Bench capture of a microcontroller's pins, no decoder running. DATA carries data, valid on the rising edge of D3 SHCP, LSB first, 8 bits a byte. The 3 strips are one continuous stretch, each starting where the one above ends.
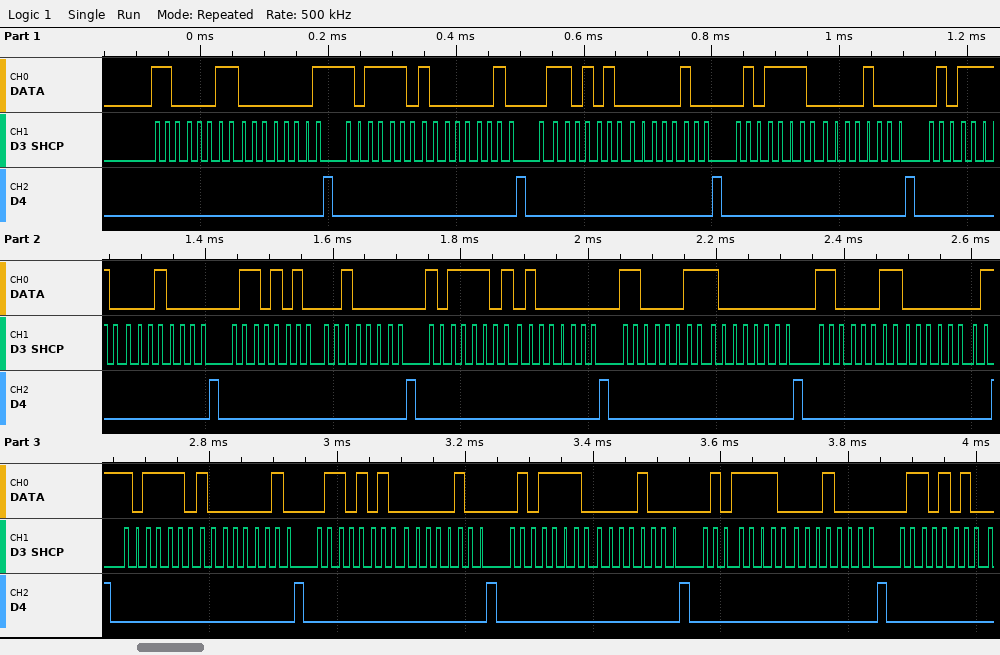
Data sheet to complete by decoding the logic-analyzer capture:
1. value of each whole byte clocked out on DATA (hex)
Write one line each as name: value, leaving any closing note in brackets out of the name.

value of each whole byte clocked out on DATA: C3 80 BD 40 56 20 7A 10 7A 08 56 04 BD 02 C3 01 C3 80 BD 40 56 20 7A 10 7A 08 56
